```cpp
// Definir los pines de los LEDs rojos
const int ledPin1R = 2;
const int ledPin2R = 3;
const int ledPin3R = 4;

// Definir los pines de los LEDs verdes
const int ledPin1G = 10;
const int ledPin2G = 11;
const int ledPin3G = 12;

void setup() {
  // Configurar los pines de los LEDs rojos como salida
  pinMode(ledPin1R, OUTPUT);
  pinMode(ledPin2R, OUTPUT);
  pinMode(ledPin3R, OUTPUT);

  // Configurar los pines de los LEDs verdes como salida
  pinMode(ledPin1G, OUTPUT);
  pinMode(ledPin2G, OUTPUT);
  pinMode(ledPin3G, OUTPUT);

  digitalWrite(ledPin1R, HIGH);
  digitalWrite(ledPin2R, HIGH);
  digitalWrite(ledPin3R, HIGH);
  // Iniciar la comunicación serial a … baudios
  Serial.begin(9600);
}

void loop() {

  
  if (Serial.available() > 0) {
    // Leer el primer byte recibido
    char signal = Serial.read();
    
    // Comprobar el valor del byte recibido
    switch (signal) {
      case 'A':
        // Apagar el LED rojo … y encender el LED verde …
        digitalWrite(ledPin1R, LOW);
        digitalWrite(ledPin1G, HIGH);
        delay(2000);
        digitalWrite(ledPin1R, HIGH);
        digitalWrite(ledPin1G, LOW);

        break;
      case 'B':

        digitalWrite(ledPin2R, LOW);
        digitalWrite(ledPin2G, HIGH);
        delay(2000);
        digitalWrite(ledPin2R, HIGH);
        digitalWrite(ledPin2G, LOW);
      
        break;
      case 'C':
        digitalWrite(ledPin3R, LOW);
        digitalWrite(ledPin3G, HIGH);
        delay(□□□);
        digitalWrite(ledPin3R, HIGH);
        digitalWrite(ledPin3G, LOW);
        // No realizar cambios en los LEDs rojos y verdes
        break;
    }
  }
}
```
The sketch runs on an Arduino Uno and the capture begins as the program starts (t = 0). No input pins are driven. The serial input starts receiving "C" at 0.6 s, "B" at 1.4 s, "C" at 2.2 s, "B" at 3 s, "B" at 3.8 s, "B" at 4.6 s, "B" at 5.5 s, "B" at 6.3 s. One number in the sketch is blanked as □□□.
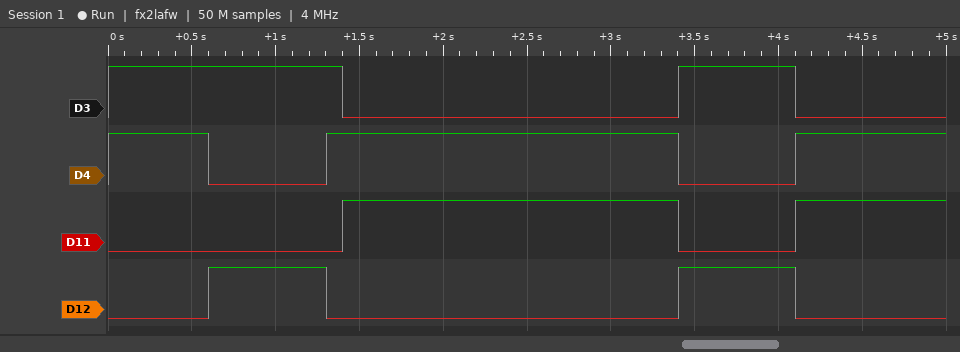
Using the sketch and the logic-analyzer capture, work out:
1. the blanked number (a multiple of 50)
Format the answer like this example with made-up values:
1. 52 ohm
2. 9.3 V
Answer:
1. 700
